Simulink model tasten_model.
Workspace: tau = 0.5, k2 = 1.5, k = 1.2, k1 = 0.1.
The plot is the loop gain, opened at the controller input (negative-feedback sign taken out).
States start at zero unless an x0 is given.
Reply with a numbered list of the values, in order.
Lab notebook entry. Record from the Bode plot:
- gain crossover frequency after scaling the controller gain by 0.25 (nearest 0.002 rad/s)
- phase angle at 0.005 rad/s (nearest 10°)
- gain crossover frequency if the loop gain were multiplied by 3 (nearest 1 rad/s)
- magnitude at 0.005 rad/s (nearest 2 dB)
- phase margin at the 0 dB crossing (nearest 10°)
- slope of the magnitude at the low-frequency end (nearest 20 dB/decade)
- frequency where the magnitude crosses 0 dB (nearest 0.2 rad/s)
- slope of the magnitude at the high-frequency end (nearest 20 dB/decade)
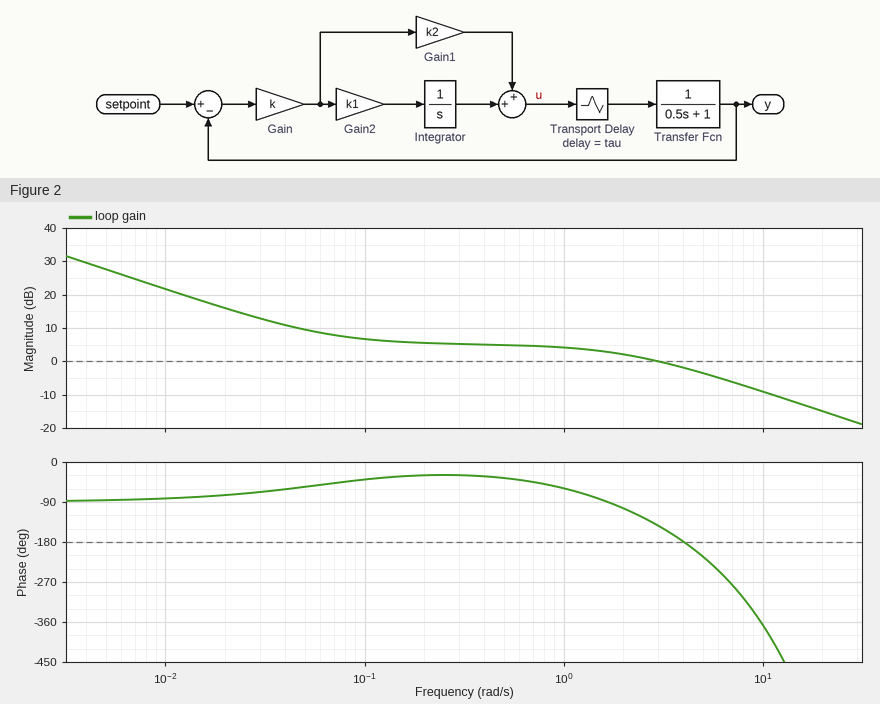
1. 0.034 rad/s
2. -90°
3. 11 rad/s
4. 28 dB
5. 40°
6. -20 dB/decade
7. 3.0 rad/s
8. -20 dB/decade
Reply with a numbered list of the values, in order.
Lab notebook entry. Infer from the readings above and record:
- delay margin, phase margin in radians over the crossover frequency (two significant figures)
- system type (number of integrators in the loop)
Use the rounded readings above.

1. 0.23 s
2. 1
